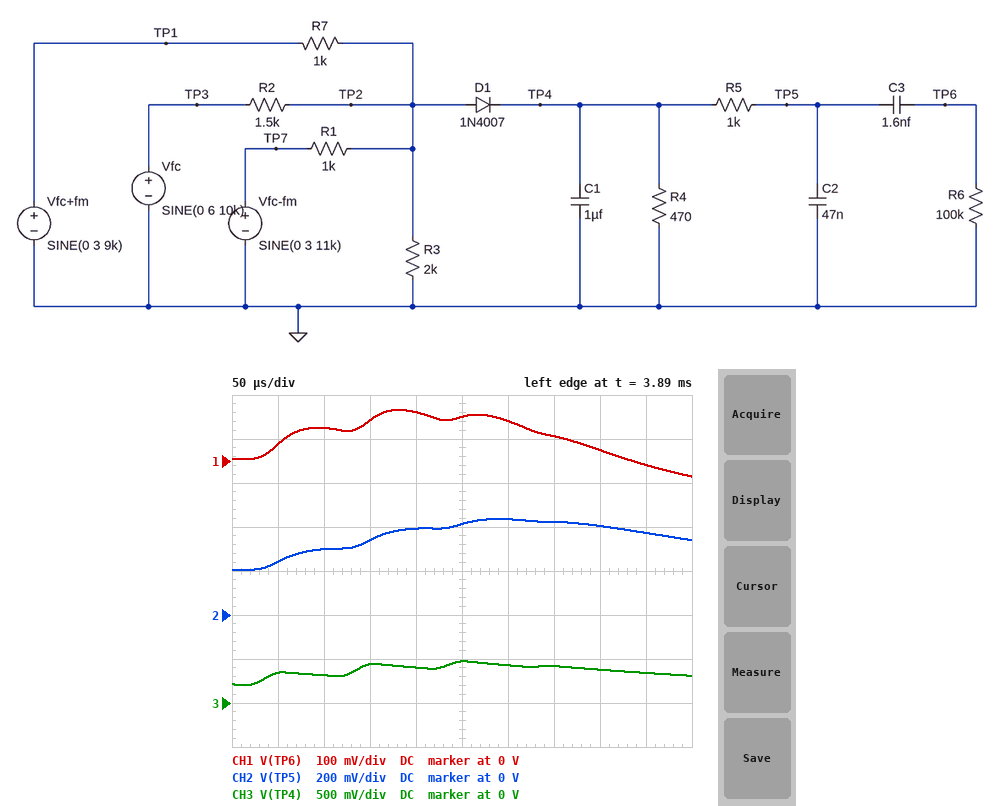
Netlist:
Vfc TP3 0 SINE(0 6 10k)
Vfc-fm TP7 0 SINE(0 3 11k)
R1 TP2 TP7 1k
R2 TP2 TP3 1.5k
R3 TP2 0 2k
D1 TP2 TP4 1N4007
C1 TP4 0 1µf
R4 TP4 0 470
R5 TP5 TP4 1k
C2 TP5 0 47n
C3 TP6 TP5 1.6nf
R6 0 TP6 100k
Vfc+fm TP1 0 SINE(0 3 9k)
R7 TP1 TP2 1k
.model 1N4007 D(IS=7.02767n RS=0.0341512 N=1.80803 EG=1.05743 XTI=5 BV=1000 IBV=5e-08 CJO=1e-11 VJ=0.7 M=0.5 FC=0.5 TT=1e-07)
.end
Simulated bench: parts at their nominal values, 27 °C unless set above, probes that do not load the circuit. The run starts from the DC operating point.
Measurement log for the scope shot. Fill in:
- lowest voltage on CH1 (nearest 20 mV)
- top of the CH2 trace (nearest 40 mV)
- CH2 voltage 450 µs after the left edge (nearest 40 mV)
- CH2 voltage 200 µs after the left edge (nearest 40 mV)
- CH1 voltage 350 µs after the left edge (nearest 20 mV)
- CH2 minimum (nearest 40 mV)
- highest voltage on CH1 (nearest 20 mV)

-40 mV
440 mV
360 mV
400 mV
60 mV
200 mV
120 mV
